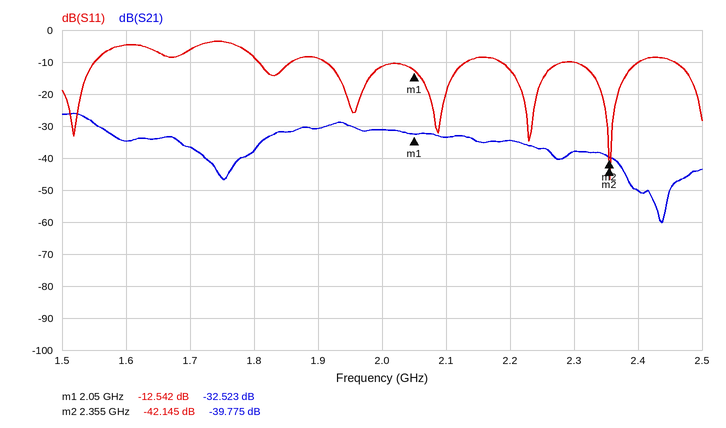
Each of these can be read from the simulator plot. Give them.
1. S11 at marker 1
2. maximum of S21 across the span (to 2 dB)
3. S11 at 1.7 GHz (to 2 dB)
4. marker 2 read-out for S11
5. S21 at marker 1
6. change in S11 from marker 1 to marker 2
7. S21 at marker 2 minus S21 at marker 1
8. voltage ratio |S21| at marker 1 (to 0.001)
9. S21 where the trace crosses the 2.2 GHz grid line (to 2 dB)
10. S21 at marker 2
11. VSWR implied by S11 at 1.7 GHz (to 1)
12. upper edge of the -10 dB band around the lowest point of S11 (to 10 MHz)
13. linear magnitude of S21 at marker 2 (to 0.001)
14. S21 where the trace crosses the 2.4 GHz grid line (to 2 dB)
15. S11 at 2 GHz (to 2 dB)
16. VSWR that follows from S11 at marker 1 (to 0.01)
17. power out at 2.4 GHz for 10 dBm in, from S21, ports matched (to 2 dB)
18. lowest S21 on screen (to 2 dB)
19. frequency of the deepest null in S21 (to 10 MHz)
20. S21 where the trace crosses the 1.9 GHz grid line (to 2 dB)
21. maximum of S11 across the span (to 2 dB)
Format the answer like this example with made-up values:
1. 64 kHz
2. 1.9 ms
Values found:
1. -12.542 dB
2. -26 dB
3. -6 dB
4. -42.145 dB
5. -32.523 dB
6. -29.603 dB
7. -7.252 dB
8. 0.024
9. -34 dB
10. -39.775 dB
11. 3
12. 2.40 GHz
13. 0.010
14. -50 dB
15. -12 dB
16. 1.62
17. -40 dBm
18. -60 dB
19. 2.44 GHz
20. -30 dB
21. -4 dB
